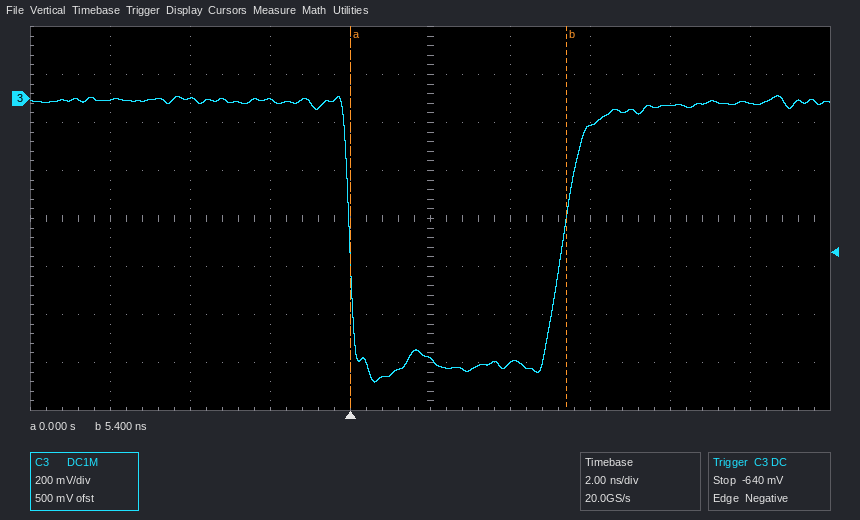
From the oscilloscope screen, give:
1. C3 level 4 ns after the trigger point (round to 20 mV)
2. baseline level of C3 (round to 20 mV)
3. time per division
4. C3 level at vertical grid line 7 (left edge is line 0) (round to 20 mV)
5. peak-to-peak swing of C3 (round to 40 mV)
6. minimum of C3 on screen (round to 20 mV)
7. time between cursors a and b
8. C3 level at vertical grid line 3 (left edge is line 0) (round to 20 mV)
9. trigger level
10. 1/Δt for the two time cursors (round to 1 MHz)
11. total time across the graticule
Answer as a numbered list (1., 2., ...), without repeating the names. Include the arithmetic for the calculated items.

1. -1.10 V
2. -20 mV
3. 2 ns
4. -120 mV
5. 1.20 V
6. -1.18 V
7. 5.4 ns − (0 s) = 5.4 ns
8. 0 mV
9. -640 mV
10. 1 / 5.4 ns ≈ 185 MHz
11. 20 ns
